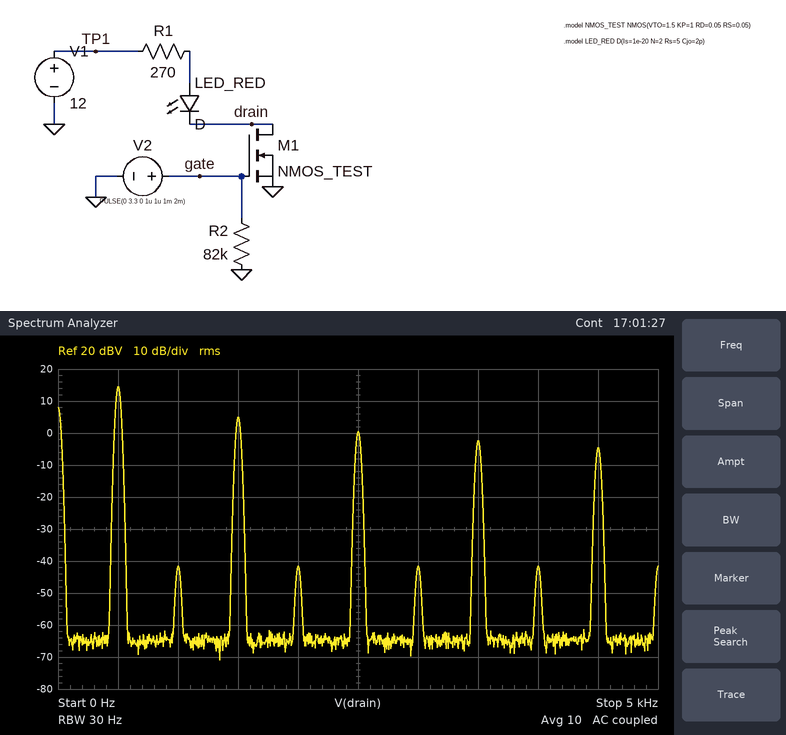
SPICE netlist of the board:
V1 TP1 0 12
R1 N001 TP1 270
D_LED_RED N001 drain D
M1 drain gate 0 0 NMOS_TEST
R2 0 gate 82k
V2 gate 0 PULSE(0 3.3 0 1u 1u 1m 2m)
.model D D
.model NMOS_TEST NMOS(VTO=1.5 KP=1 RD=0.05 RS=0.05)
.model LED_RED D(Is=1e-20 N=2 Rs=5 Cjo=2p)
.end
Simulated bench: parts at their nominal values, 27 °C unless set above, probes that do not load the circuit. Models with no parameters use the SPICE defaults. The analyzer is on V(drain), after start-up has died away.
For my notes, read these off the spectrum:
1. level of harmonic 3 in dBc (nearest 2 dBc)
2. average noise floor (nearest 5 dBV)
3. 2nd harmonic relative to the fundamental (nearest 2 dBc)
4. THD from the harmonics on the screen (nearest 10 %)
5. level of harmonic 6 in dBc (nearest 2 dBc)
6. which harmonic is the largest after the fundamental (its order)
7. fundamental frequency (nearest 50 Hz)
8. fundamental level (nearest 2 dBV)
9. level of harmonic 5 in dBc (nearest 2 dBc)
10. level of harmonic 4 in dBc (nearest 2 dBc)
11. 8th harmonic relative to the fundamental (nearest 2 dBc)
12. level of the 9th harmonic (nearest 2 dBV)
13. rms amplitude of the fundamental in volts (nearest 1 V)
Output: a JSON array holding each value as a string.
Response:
["-10 dBc", "-65 dBV", "-56 dBc", "40 %", "-56 dBc", "3", "500 Hz", "14 dBV", "-14 dBc", "-56 dBc", "-56 dBc", "-4 dBV", "5 V"]
